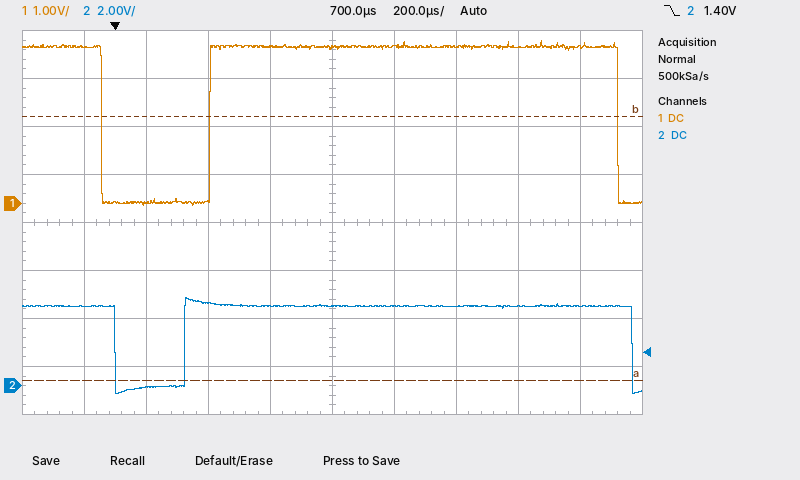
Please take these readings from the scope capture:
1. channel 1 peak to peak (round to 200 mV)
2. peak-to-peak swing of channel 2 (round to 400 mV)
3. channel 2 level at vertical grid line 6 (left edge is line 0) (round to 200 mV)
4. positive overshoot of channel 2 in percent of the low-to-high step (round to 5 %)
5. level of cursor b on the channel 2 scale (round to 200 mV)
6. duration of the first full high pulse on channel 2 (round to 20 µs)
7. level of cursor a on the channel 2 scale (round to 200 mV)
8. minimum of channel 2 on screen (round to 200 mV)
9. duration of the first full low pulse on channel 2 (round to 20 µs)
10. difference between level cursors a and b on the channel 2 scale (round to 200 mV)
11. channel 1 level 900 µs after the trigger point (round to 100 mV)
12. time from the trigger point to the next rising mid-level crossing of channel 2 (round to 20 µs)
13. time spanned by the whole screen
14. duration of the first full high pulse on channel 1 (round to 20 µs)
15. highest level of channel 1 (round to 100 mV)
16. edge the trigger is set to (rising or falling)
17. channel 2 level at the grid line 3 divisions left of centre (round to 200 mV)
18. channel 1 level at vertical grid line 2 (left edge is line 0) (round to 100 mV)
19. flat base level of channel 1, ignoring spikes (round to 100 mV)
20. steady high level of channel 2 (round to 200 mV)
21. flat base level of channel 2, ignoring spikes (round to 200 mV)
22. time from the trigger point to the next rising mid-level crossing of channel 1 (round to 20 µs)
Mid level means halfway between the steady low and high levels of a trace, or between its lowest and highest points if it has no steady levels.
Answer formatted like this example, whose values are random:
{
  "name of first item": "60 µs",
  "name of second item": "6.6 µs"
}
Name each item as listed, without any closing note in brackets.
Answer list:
{
  "channel 1 peak to peak": "3.4 V",
  "peak-to-peak swing of channel 2": "4.0 V",
  "channel 2 level at vertical grid line 6 (left edge is line 0)": "3.4 V",
  "positive overshoot of channel 2 in percent of the low-to-high step": "10 %",
  "level of cursor b on the channel 2 scale": "11.2 V",
  "duration of the first full high pulse on channel 2": "1.44 ms",
  "level of cursor a on the channel 2 scale": "200 mV",
  "minimum of channel 2 on screen": "-400 mV",
  "duration of the first full low pulse on channel 2": "220 µs",
  "difference between level cursors a and b on the channel 2 scale": "11.0 V",
  "channel 1 level 900 µs after the trigger point": "3.3 V",
  "time from the trigger point to the next rising mid-level crossing of channel 2": "220 µs",
  "time spanned by the whole screen": "2 ms",
  "duration of the first full high pulse on channel 1": "1.32 ms",
  "highest level of channel 1": "3.4 V",
  "edge the trigger is set to": "falling",
  "channel 2 level at the grid line 3 divisions left of centre": "0.0 V",
  "channel 1 level at vertical grid line 2 (left edge is line 0)": "0.0 V",
  "flat base level of channel 1, ignoring spikes": "0.0 V",
  "steady high level of channel 2": "3.4 V",
  "flat base level of channel 2, ignoring spikes": "0.0 V",
  "time from the trigger point to the next rising mid-level crossing of channel 1": "300 µs"
}
